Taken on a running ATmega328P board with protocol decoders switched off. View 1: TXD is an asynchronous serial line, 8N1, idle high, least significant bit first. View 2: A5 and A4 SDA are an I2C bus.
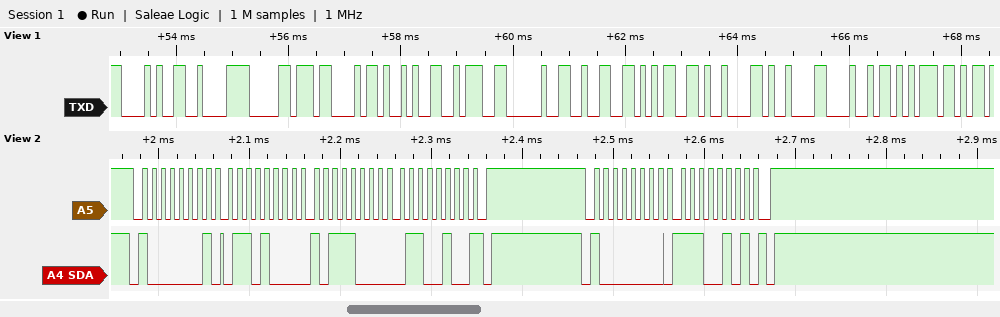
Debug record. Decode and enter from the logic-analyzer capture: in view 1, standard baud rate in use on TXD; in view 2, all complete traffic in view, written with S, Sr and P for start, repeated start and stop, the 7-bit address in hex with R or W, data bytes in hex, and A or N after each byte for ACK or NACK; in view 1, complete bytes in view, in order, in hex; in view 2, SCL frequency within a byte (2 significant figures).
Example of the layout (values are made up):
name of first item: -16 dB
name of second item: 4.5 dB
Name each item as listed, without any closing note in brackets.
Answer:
in view 1, standard baud rate in use on TXD: 9600 baud
in view 2, all complete traffic in view, written with S, Sr and P for start, repeated start and stop, the 7-bit address in hex with R or W, data bytes in hex, and A or N after each byte for ACK or NACK: S 40R A 68 A B8 A 64 N P S 40W A E5 A P
in view 1, complete bytes in view, in order, in hex: 0x28 0xC2 0xB0 0x43 0x29 0x3A 0x20 0x32 0x35 0x09 0x09 0x48 0x75
in view 2, SCL frequency within a byte: 100 kHz
